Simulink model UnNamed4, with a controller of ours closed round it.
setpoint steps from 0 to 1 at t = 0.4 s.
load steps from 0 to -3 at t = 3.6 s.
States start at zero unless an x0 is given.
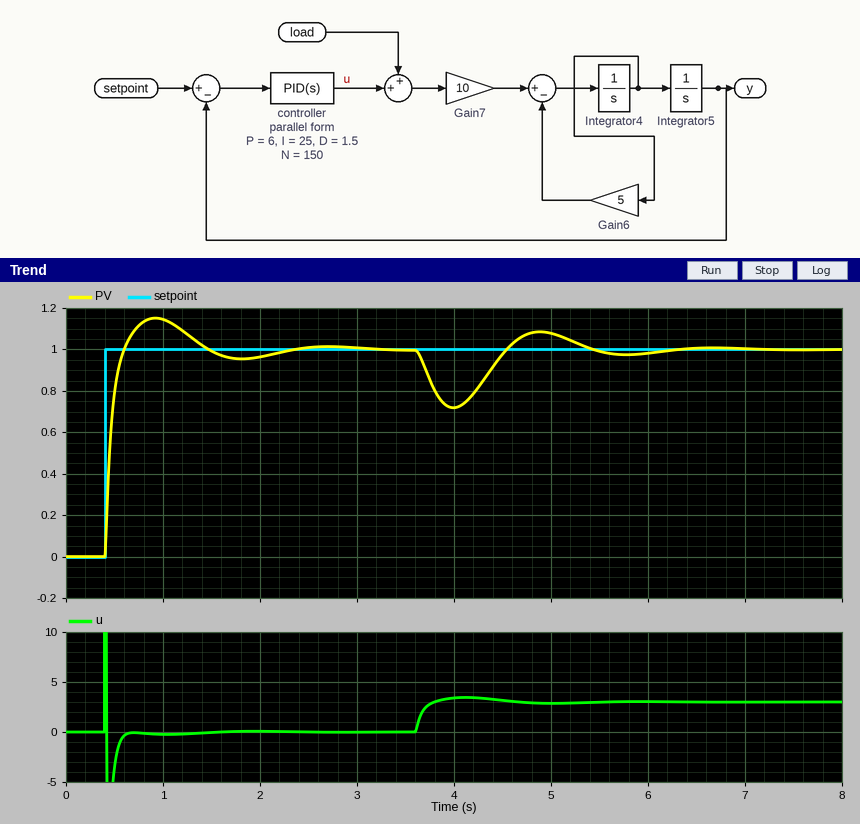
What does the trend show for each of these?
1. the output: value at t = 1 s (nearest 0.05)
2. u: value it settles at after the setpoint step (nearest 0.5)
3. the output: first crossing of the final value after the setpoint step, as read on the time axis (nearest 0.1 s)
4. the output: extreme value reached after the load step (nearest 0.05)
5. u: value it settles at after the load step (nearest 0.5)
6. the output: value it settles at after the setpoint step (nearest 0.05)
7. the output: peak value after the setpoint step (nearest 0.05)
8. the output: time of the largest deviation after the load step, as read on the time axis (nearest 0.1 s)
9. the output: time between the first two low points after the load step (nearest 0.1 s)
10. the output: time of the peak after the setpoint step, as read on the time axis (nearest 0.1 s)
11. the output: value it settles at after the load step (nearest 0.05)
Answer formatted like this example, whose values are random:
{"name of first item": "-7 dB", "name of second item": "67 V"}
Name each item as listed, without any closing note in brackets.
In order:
{"the output: value at t = 1 s": "1.15", "u: value it settles at after the setpoint step": "0.0", "the output: first crossing of the final value after the setpoint step, as read on the time axis": "0.6 s", "the output: extreme value reached after the load step": "0.70", "u: value it settles at after the load step": "3.0", "the output: value it settles at after the setpoint step": "1.00", "the output: peak value after the setpoint step": "1.15", "the output: time of the largest deviation after the load step, as read on the time axis": "4.0 s", "the output: time between the first two low points after the load step": "1.8 s", "the output: time of the peak after the setpoint step, as read on the time axis": "0.9 s", "the output: value it settles at after the load step": "1.00"}
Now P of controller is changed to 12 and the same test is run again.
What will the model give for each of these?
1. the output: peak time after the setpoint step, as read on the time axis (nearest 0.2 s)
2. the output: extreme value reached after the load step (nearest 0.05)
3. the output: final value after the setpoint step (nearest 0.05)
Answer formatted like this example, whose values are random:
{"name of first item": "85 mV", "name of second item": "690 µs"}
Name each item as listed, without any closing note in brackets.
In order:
{"the output: peak time after the setpoint step, as read on the time axis": "0.6 s", "the output: extreme value reached after the load step": "0.80", "the output: final value after the setpoint step": "1.00"}
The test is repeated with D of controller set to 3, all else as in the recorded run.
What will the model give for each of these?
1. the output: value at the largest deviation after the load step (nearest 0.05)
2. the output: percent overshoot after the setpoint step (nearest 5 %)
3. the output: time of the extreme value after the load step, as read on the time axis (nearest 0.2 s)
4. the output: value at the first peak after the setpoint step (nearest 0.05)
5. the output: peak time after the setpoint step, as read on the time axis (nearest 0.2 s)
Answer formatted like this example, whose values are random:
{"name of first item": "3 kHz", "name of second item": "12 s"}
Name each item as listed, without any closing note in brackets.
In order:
{"the output: value at the largest deviation after the load step": "0.80", "the output: percent overshoot after the setpoint step": "10 %", "the output: time of the extreme value after the load step, as read on the time axis": "4.2 s", "the output: value at the first peak after the setpoint step": "1.10", "the output: peak time after the setpoint step, as read on the time axis": "1.2 s"}
